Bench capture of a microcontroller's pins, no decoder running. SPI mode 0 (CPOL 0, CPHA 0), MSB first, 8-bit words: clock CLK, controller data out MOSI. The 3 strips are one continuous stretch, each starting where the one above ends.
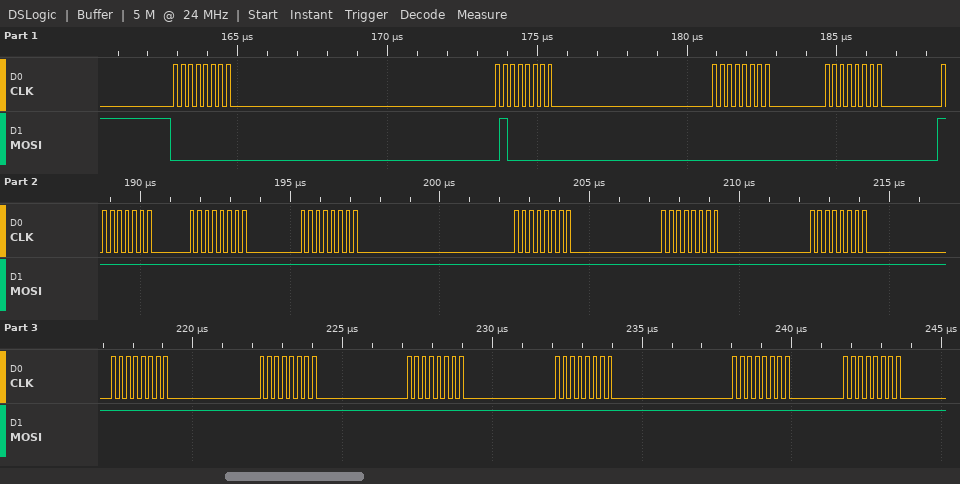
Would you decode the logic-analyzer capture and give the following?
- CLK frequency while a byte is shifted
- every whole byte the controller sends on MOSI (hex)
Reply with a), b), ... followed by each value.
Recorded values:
a) 4 MHz
b) 00 40 00 00 FF FF FF FF FF FF FF FF FF FF FF FF
